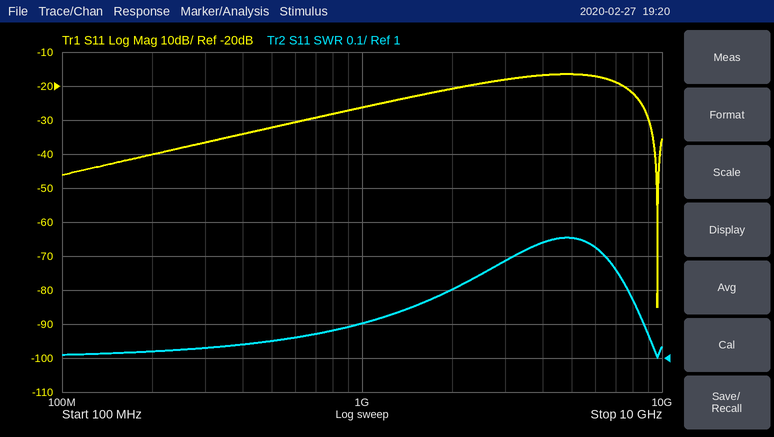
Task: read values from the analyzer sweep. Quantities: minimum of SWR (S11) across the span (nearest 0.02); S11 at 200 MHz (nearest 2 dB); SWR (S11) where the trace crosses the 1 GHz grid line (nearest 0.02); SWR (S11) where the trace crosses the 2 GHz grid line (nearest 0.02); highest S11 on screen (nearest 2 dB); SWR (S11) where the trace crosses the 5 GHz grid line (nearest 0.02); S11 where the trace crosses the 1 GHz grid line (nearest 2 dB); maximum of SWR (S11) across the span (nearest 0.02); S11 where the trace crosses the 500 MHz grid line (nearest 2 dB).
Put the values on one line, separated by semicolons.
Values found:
1.00; -40 dB; 1.10; 1.20; -16 dB; 1.36; -26 dB; 1.36; -32 dB
